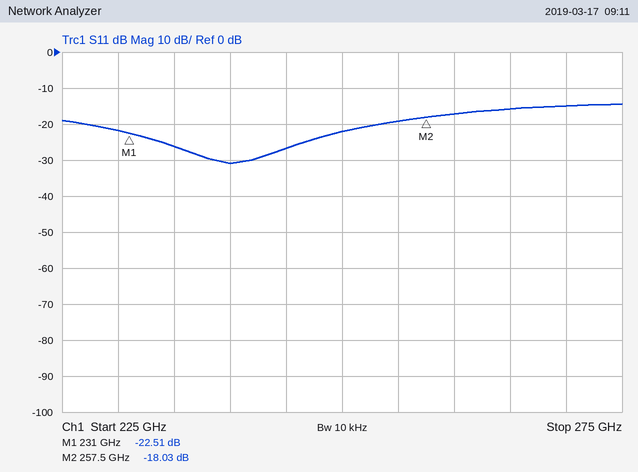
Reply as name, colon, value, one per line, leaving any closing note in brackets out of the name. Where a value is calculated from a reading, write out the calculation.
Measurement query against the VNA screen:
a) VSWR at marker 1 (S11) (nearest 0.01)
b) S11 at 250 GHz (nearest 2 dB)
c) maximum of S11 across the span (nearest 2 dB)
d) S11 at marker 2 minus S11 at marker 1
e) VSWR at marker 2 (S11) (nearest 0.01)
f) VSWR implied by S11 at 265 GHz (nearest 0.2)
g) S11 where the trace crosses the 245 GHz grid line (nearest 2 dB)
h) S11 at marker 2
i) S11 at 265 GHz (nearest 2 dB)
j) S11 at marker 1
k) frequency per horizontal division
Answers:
VSWR at marker 1 (S11): (1 + 0.0749)/(1 − 0.0749) ≈ 1.16
S11 at 250 GHz: -22 dB
maximum of S11 across the span: -14 dB
S11 at marker 2 minus S11 at marker 1: -18.03 − (-22.51) = 4.48 dB
VSWR at marker 2 (S11): (1 + 0.1255)/(1 − 0.1255) ≈ 1.29
VSWR implied by S11 at 265 GHz: |Γ| = 10^(-16/20) = 0.1585; VSWR = (1 + 0.1585)/(1 − 0.1585) ≈ 1.4
S11 where the trace crosses the 245 GHz grid line: -26 dB
S11 at marker 2: -18.03 dB
S11 at 265 GHz: -16 dB
S11 at marker 1: -22.51 dB
frequency per horizontal division: 5 GHz
